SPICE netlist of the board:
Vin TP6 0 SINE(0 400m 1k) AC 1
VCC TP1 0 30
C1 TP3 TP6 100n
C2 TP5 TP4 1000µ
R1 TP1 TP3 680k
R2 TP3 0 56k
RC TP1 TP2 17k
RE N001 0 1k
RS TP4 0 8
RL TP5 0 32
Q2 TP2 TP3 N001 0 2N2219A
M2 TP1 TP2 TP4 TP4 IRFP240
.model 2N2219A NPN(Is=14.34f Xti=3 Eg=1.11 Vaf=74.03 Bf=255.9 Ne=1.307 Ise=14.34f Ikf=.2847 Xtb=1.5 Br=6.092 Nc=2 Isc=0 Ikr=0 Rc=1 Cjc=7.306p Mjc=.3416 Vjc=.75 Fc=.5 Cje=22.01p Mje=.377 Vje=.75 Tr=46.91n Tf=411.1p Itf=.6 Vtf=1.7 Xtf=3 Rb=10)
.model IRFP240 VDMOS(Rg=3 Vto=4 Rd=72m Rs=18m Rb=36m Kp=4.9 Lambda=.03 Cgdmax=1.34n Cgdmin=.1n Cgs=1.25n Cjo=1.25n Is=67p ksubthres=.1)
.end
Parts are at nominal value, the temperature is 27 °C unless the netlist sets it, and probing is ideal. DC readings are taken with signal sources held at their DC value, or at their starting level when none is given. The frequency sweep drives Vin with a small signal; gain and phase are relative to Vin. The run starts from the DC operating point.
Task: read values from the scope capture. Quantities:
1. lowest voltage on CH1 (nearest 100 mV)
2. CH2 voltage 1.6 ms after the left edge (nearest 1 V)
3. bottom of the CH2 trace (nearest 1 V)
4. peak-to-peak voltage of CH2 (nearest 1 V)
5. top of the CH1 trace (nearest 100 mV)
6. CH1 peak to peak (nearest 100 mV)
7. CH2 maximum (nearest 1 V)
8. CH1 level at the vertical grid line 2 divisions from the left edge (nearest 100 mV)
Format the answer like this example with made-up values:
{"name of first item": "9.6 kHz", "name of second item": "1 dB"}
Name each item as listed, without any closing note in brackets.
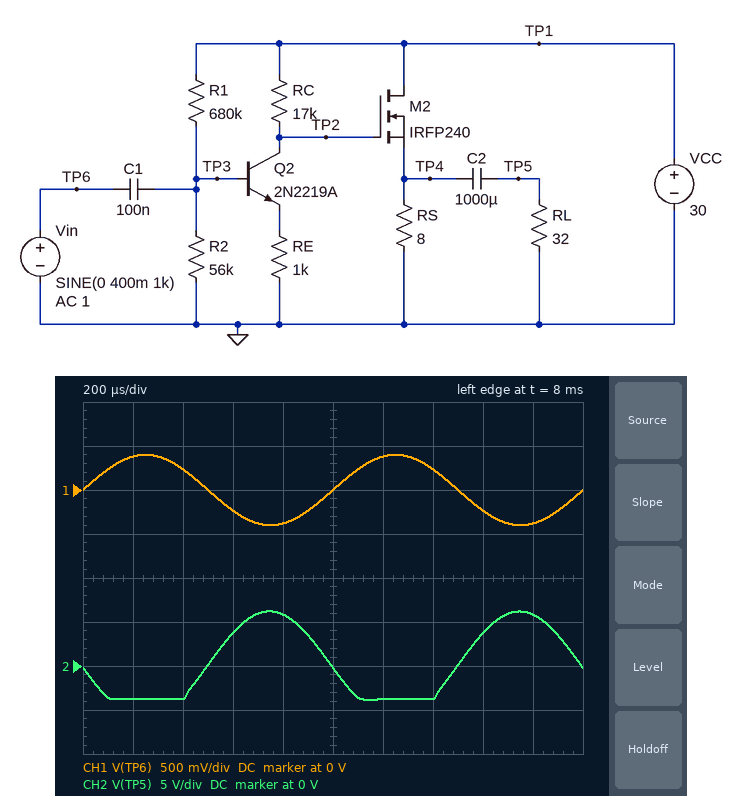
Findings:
{"lowest voltage on CH1": "-400 mV", "CH2 voltage 1.6 ms after the left edge": "4 V", "bottom of the CH2 trace": "-4 V", "peak-to-peak voltage of CH2": "10 V", "top of the CH1 trace": "400 mV", "CH1 peak to peak": "800 mV", "CH2 maximum": "6 V", "CH1 level at the vertical grid line 2 divisions from the left edge": "200 mV"}
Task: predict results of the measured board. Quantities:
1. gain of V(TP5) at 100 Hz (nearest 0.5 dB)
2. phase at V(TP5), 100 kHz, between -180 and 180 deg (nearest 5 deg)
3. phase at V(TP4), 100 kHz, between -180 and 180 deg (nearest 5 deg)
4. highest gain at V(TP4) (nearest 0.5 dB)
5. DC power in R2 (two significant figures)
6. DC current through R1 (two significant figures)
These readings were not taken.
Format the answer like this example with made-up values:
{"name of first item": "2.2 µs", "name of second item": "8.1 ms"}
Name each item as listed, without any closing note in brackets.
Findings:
{"gain of V(TP5) at 100 Hz": "23.0 dB", "phase at V(TP5), 100 kHz, between -180 and 180 deg": "115 deg", "phase at V(TP4), 100 kHz, between -180 and 180 deg": "115 deg", "highest gain at V(TP4)": "24.0 dB", "DC power in R2": "64 µW", "DC current through R1": "41 µA"}
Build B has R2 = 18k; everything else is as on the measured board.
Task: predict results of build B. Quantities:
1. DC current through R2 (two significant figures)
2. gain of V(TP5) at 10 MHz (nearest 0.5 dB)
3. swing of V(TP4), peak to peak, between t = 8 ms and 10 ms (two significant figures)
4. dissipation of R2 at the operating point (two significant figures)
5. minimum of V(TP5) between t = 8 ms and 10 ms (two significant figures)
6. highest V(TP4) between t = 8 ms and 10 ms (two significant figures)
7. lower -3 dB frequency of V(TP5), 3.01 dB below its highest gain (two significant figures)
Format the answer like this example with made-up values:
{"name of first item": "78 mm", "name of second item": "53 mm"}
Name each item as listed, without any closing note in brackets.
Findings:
{"DC current through R2": "42 µA", "gain of V(TP5) at 10 MHz": "-28.0 dB", "swing of V(TP4), peak to peak, between t = 8 ms and 10 ms": "8.5 V", "dissipation of R2 at the operating point": "32 µW", "minimum of V(TP5) between t = 8 ms and 10 ms": "-5.7 V", "highest V(TP4) between t = 8 ms and 10 ms": "25 V", "lower -3 dB frequency of V(TP5), 3.01 dB below its highest gain": "98 Hz"}
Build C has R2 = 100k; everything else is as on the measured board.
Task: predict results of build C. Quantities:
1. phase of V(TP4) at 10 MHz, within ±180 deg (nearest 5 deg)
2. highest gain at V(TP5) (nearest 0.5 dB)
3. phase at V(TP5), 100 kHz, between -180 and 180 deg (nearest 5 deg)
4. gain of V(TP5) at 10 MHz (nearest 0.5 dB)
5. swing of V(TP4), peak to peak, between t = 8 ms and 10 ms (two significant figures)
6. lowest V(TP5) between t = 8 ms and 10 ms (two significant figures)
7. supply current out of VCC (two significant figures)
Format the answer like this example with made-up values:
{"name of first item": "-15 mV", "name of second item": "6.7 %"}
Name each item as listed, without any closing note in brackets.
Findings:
{"phase of V(TP4) at 10 MHz, within ±180 deg": "85 deg", "highest gain at V(TP5)": "-18.0 dB", "phase at V(TP5), 100 kHz, between -180 and 180 deg": "-165 deg", "gain of V(TP5) at 10 MHz": "-31.0 dB", "swing of V(TP4), peak to peak, between t = 8 ms and 10 ms": "8.4 V", "lowest V(TP5) between t = 8 ms and 10 ms": "-650 mV", "supply current out of VCC": "1.7 mA"}
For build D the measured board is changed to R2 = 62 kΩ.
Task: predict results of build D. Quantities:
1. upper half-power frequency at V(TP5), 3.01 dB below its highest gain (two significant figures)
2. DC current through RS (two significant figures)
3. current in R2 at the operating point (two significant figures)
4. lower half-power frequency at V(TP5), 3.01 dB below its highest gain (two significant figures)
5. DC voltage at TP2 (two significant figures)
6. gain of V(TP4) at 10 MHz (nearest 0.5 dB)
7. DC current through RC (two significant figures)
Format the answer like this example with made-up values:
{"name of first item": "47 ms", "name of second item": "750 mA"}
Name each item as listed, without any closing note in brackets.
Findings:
{"upper half-power frequency at V(TP5), 3.01 dB below its highest gain": "45 kHz", "DC current through RS": "320 mA", "current in R2 at the operating point": "33 µA", "lower half-power frequency at V(TP5), 3.01 dB below its highest gain": "40 Hz", "DC voltage at TP2": "6.8 V", "gain of V(TP4) at 10 MHz": "-23.0 dB", "DC current through RC": "1.4 mA"}
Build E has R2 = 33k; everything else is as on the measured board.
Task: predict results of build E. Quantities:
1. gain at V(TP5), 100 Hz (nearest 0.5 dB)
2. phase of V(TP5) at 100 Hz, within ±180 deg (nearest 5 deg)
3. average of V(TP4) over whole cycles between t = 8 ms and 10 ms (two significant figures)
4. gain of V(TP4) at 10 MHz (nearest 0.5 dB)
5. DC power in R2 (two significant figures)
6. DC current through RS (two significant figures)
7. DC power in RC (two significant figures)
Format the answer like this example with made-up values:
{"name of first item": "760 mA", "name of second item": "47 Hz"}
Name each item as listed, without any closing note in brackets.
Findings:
{"gain at V(TP5), 100 Hz": "22.5 dB", "phase of V(TP5) at 100 Hz, within ±180 deg": "-145 deg", "average of V(TP4) over whole cycles between t = 8 ms and 10 ms": "14 V", "gain of V(TP4) at 10 MHz": "-22.5 dB", "DC power in R2": "49 µW", "DC current through RS": "1.8 A", "DC power in RC": "6.9 mW"}
